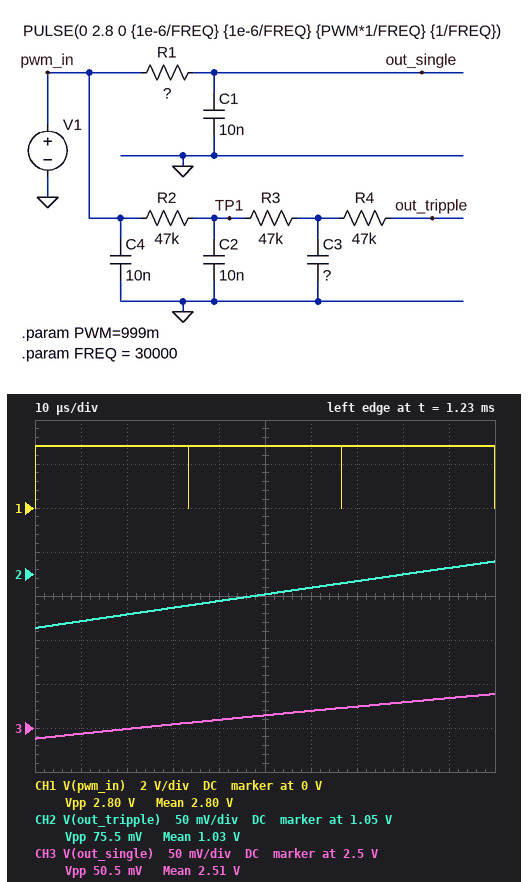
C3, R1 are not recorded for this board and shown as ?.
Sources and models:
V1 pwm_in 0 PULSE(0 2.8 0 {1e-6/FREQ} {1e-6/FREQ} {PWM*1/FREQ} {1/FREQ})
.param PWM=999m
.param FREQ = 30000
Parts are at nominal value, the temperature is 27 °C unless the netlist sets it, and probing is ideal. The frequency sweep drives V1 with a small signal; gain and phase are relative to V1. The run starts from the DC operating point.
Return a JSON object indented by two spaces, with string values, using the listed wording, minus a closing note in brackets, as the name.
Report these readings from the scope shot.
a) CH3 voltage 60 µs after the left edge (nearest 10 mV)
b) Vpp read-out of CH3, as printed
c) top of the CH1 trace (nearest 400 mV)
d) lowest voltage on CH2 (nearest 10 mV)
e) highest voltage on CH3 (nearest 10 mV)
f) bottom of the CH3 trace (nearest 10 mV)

{
  "CH3 voltage 60 µs after the left edge": "2.52 V",
  "Vpp read-out of CH3, as printed": "50.5 mV",
  "top of the CH1 trace": "2.8 V",
  "lowest voltage on CH2": "990 mV",
  "highest voltage on CH3": "2.54 V",
  "bottom of the CH3 trace": "2.49 V"
}
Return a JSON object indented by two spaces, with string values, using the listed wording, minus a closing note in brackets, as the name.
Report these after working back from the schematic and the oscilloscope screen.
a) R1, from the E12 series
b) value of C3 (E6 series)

{
  "R1, from the E12 series": "56 kΩ",
  "value of C3": "22 nF"
}
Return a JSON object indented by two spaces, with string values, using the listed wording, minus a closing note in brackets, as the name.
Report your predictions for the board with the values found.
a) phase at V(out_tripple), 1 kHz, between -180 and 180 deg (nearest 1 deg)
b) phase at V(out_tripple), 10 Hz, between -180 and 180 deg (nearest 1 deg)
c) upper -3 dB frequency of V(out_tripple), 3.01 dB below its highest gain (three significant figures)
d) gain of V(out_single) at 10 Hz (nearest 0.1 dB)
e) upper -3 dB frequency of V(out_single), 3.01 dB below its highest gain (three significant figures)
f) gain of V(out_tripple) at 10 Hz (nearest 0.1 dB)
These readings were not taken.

{
  "phase at V(out_tripple), 1 kHz, between -180 and 180 deg": "-139 deg",
  "phase at V(out_tripple), 10 Hz, between -180 and 180 deg": "-9 deg",
  "upper -3 dB frequency of V(out_tripple), 3.01 dB below its highest gain": "67.8 Hz",
  "gain of V(out_single) at 10 Hz": "0 dB",
  "upper -3 dB frequency of V(out_single), 3.01 dB below its highest gain": "284 Hz",
  "gain of V(out_tripple) at 10 Hz": "-0.1 dB"
}
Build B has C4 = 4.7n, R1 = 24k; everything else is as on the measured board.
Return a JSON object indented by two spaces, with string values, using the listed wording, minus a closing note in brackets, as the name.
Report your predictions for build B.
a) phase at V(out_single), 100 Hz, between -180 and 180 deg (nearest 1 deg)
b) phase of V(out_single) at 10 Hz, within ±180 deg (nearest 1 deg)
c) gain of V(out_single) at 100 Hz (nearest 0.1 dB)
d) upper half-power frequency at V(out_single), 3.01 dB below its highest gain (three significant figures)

{
  "phase at V(out_single), 100 Hz, between -180 and 180 deg": "-9 deg",
  "phase of V(out_single) at 10 Hz, within ±180 deg": "-1 deg",
  "gain of V(out_single) at 100 Hz": "-0.1 dB",
  "upper half-power frequency at V(out_single), 3.01 dB below its highest gain": "663 Hz"
}
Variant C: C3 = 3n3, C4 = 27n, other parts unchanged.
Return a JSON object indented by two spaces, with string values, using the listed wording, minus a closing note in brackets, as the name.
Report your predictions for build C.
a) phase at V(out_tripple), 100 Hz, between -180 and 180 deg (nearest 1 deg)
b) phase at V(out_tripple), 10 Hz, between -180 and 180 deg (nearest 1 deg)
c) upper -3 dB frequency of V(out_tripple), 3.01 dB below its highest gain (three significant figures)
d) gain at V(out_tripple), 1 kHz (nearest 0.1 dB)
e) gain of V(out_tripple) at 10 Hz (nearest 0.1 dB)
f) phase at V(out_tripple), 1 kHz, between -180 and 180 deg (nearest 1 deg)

{
  "phase at V(out_tripple), 100 Hz, between -180 and 180 deg": "-27 deg",
  "phase at V(out_tripple), 10 Hz, between -180 and 180 deg": "-3 deg",
  "upper -3 dB frequency of V(out_tripple), 3.01 dB below its highest gain": "231 Hz",
  "gain at V(out_tripple), 1 kHz": "-14.4 dB",
  "gain of V(out_tripple) at 10 Hz": "0 dB",
  "phase at V(out_tripple), 1 kHz, between -180 and 180 deg": "-111 deg"
}
